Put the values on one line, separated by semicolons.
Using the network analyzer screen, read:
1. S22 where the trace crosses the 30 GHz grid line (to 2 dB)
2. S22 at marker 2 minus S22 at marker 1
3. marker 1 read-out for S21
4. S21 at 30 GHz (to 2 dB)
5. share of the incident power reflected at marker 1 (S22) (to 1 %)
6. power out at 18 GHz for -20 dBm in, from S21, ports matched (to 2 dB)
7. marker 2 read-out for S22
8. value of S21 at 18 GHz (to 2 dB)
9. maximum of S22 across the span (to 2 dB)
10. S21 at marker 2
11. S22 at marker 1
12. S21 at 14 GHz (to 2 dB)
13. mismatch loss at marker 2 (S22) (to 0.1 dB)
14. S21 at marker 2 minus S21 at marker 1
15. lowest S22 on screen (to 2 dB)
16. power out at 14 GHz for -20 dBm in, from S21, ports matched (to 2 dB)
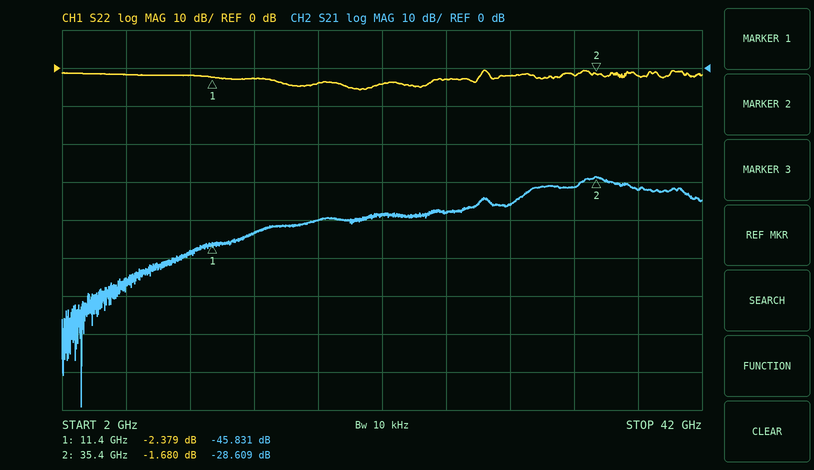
-2 dB; 0.699 dB; -45.831 dB; -36 dB; 58 %; -60 dBm; -1.680 dB; -40 dB; 0 dB; -28.609 dB; -2.379 dB; -44 dB; 4.9 dB; 17.222 dB; -6 dB; -64 dBm
